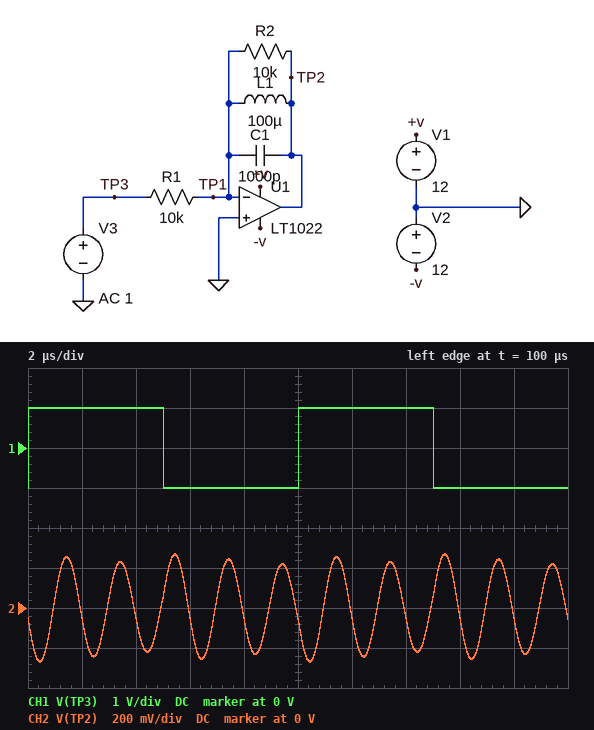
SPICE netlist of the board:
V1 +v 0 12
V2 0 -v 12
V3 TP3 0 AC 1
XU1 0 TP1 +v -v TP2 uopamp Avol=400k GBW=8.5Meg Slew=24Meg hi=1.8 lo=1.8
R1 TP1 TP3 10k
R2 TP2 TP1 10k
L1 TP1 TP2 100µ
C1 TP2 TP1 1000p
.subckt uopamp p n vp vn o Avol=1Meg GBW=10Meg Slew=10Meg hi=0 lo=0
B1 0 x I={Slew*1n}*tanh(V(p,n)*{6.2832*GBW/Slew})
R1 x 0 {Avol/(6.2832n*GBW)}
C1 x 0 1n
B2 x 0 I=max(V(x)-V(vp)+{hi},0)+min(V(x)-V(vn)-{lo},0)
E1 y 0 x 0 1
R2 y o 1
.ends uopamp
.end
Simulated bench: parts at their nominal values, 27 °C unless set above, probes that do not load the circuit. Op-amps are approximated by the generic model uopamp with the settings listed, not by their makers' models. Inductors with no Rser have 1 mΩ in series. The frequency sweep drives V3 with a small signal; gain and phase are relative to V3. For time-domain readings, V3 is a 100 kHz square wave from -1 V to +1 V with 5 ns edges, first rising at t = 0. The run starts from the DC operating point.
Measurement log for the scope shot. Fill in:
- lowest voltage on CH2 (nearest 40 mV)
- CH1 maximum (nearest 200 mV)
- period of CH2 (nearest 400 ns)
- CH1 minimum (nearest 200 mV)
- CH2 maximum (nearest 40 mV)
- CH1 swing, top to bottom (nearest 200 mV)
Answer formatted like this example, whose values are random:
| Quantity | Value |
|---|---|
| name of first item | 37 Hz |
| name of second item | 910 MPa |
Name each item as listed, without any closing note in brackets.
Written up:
| Quantity | Value |
|---|---|
| lowest voltage on CH2 | -280 mV |
| CH1 maximum | 1.0 V |
| period of CH2 | 2.0 µs |
| CH1 minimum | -1.0 V |
| CH2 maximum | 280 mV |
| CH1 swing, top to bottom | 2.0 V |
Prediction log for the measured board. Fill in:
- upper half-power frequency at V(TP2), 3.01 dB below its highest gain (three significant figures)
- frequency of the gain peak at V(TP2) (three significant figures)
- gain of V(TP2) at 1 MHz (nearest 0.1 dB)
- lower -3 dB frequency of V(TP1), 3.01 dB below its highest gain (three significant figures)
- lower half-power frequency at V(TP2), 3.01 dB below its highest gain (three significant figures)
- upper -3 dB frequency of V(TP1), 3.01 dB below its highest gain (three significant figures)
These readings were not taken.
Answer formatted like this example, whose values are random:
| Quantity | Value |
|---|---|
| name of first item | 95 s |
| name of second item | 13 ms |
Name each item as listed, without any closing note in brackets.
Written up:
| Quantity | Value |
|---|---|
| upper half-power frequency at V(TP2), 3.01 dB below its highest gain | 511 kHz |
| frequency of the gain peak at V(TP2) | 503 kHz |
| gain of V(TP2) at 1 MHz | -33.5 dB |
| lower -3 dB frequency of V(TP1), 3.01 dB below its highest gain | 495 kHz |
| lower half-power frequency at V(TP2), 3.01 dB below its highest gain | 495 kHz |
| upper -3 dB frequency of V(TP1), 3.01 dB below its highest gain | 511 kHz |
